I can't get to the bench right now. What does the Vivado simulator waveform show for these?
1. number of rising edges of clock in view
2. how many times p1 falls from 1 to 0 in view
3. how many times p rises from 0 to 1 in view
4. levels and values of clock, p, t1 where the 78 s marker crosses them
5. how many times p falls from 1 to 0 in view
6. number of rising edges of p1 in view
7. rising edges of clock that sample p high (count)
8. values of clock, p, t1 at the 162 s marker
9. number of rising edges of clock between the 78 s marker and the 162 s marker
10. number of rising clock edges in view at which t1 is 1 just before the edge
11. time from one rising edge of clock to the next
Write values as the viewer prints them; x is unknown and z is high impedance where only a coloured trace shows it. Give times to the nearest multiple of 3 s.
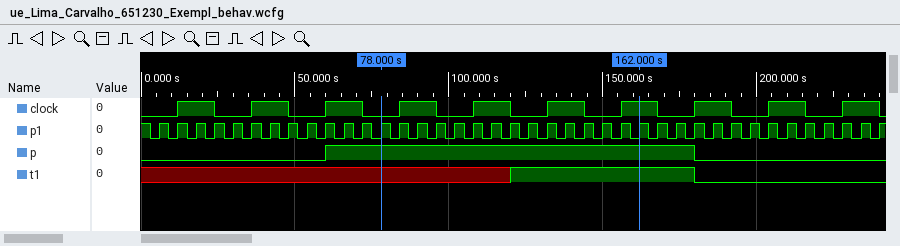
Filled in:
10
40
1
clock=0, p=1, t1=x
1
40
5
clock=1, p=1, t1=1
4
3
24 s
